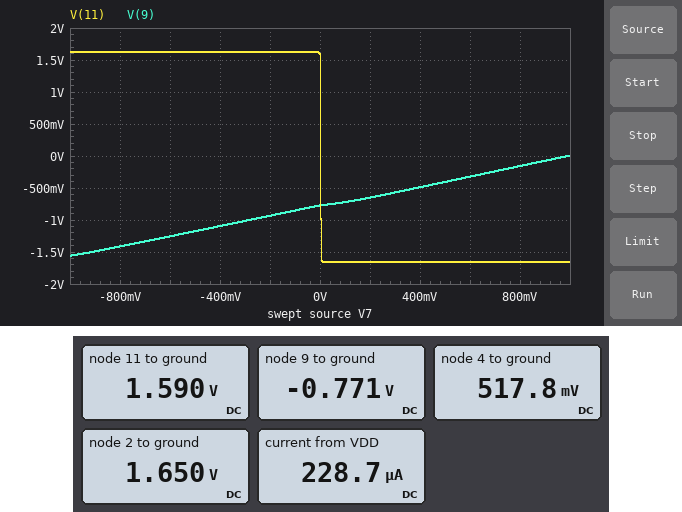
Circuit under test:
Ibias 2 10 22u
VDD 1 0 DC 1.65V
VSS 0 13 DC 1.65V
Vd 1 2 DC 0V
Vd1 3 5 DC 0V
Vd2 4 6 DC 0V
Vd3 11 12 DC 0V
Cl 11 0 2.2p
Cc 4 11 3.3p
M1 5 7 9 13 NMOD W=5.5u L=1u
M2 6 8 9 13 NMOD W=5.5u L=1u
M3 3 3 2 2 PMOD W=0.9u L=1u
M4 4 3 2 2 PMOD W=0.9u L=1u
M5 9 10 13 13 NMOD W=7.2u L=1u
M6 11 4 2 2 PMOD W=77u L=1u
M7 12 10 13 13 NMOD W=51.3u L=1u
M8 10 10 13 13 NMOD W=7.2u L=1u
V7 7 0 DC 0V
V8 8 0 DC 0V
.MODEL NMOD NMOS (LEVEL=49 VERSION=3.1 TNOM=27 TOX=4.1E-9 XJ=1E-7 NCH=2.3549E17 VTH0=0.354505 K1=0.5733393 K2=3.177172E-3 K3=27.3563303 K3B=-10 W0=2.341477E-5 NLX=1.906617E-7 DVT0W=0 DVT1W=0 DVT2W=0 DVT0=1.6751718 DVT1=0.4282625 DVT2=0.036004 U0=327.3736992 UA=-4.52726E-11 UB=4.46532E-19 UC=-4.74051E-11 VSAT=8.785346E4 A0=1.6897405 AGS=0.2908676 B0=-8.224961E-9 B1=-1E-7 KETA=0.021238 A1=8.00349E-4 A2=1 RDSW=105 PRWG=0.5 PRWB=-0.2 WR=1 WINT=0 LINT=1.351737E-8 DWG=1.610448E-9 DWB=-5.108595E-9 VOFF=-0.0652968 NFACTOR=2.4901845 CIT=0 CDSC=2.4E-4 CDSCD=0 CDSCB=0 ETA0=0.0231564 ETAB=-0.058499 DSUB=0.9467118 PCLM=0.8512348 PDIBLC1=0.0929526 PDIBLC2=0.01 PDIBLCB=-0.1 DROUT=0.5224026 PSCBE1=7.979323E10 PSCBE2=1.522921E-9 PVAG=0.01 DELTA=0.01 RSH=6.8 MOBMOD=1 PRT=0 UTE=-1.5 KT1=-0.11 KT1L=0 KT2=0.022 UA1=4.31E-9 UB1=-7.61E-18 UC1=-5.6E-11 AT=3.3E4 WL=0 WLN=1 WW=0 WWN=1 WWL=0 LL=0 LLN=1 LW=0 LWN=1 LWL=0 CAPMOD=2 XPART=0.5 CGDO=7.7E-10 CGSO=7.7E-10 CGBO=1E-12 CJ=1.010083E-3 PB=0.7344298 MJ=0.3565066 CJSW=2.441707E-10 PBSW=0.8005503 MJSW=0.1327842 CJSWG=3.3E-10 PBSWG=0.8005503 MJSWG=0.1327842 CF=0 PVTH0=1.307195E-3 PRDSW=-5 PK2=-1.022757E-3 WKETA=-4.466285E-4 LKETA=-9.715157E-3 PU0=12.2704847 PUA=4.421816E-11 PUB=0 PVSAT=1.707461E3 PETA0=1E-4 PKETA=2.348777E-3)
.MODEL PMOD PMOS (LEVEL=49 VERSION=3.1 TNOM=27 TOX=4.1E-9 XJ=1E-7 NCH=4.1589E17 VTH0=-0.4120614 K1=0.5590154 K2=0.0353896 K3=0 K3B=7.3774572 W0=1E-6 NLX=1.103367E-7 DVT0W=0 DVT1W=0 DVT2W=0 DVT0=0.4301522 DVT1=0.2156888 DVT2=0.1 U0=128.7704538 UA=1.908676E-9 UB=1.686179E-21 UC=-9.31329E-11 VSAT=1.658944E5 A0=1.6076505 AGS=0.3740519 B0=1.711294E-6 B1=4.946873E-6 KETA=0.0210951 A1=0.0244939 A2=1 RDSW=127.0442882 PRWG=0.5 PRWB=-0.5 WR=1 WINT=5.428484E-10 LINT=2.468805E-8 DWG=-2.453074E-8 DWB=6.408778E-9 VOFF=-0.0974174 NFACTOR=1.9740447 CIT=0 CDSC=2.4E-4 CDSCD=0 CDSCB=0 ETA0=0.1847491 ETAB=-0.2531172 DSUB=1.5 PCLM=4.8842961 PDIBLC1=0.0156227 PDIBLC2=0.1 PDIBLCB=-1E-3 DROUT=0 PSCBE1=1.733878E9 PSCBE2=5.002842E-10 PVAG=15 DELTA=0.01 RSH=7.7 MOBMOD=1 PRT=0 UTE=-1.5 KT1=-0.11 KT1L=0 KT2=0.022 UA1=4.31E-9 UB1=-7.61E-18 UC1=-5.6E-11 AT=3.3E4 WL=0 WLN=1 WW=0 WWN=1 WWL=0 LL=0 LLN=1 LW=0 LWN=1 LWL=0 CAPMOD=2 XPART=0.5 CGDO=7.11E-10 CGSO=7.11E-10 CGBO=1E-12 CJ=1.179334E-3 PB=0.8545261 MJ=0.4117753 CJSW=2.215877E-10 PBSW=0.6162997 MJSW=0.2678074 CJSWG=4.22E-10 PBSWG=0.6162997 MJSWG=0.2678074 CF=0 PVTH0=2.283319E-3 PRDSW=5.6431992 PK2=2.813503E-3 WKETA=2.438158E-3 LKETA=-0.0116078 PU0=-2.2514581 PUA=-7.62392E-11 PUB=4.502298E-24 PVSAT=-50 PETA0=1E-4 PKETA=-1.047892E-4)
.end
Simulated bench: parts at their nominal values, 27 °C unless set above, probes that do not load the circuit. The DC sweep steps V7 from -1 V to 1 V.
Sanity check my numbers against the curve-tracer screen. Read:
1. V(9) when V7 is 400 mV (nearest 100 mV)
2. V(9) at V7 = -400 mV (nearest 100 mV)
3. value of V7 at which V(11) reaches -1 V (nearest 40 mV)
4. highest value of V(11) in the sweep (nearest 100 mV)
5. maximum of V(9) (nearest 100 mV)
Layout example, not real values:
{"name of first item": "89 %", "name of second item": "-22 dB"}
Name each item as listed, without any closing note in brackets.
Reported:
{"V(9) when V7 is 400 mV": "-500 mV", "V(9) at V7 = -400 mV": "-1.1 V", "value of V7 at which V(11) reaches -1 V": "0 V", "highest value of V(11) in the sweep": "1.6 V", "maximum of V(9)": "0 V"}
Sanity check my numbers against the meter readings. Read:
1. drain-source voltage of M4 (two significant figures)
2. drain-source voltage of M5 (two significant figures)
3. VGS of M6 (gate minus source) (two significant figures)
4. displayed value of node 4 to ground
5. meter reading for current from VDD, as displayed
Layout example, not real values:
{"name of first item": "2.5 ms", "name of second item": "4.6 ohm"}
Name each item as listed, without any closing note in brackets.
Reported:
{"drain-source voltage of M4": "-1.1 V", "drain-source voltage of M5": "880 mV", "VGS of M6 (gate minus source)": "-1.1 V", "displayed value of node 4 to ground": "517.8 mV", "meter reading for current from VDD, as displayed": "228.7 µA"}
